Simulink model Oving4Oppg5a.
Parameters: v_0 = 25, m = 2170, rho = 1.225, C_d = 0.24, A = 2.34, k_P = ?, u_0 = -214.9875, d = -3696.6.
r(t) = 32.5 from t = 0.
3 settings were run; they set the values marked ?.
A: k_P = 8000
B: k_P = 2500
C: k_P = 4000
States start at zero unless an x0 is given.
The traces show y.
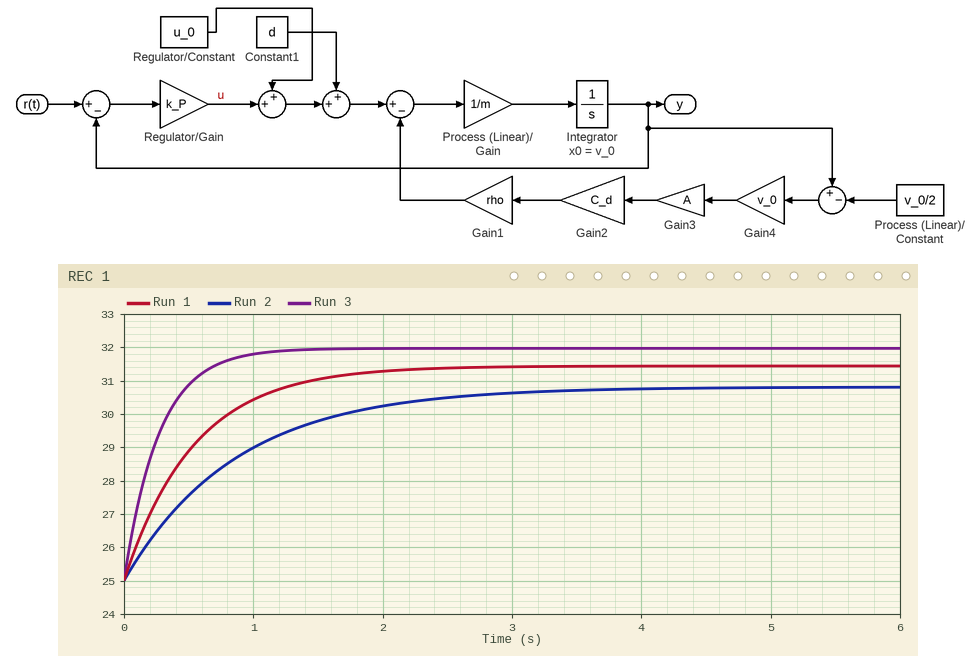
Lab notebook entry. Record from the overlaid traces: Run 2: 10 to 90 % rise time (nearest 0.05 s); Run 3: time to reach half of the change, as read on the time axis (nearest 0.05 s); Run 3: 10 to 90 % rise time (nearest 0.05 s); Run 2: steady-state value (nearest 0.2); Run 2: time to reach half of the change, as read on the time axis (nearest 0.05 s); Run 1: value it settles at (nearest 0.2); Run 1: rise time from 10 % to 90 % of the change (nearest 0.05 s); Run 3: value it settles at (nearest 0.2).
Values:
1.90 s
0.20 s
0.60 s
30.8
0.60 s
31.4
1.20 s
32.0
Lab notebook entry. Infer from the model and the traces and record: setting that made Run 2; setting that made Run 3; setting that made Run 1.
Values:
B
A
C
